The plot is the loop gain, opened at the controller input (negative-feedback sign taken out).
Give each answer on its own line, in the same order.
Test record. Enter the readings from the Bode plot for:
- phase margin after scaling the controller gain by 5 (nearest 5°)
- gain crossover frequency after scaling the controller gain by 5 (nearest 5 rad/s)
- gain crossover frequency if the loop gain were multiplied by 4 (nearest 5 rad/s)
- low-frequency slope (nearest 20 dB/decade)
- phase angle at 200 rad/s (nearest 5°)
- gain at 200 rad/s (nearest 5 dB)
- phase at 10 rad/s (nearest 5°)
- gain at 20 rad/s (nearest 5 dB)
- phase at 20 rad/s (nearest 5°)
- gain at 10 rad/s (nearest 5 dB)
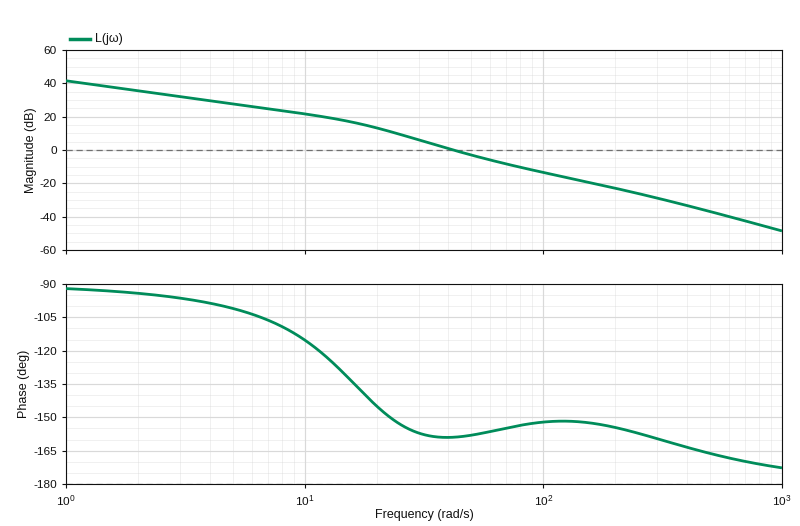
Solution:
30°
105 rad/s
90 rad/s
-20 dB/decade
-155°
-25 dB
-115°
15 dB
-145°
20 dB
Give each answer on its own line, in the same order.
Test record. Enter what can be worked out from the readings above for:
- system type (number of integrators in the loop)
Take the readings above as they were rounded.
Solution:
1
